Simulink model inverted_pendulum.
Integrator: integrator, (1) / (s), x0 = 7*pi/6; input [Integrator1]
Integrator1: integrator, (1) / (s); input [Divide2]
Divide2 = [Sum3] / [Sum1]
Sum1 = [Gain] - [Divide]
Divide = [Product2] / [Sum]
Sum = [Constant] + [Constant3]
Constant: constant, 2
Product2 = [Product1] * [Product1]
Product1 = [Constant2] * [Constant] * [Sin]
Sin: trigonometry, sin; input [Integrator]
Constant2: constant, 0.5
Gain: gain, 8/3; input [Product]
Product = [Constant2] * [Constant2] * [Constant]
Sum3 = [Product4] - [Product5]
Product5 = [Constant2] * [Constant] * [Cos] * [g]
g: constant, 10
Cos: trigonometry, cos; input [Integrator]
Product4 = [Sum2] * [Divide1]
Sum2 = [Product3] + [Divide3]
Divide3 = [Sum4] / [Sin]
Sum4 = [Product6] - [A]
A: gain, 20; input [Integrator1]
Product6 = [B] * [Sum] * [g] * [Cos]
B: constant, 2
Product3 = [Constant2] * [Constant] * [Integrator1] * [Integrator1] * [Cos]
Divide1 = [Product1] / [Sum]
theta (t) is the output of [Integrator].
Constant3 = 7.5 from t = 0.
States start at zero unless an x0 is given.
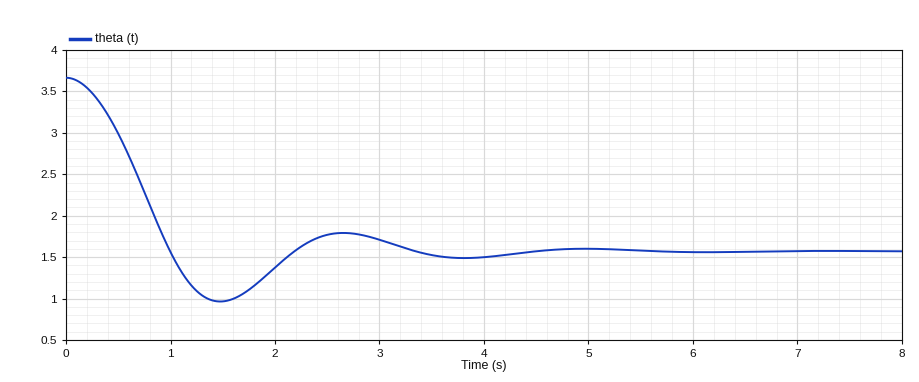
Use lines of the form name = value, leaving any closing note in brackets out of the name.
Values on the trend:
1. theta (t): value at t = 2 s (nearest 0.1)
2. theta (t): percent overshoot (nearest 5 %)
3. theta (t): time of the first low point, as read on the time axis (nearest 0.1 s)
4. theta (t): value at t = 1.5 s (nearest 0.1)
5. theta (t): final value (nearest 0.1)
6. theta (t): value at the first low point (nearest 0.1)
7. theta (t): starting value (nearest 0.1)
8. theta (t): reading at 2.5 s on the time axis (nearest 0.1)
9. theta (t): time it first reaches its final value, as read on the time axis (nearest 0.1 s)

theta (t): value at t = 2 s = 1.4
theta (t): percent overshoot = 30 %
theta (t): time of the first low point, as read on the time axis = 1.5 s
theta (t): value at t = 1.5 s = 1.0
theta (t): final value = 1.6
theta (t): value at the first low point = 1.0
theta (t): starting value = 3.7
theta (t): reading at 2.5 s on the time axis = 1.8
theta (t): time it first reaches its final value, as read on the time axis = 1.0 s
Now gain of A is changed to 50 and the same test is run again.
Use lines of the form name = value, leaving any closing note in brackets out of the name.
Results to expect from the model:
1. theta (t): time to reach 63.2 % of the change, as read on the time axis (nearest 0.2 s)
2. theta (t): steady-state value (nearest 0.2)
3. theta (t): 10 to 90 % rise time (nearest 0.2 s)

theta (t): time to reach 63.2 % of the change, as read on the time axis = 1.0 s
theta (t): steady-state value = 1.6
theta (t): 10 to 90 % rise time = 1.2 s
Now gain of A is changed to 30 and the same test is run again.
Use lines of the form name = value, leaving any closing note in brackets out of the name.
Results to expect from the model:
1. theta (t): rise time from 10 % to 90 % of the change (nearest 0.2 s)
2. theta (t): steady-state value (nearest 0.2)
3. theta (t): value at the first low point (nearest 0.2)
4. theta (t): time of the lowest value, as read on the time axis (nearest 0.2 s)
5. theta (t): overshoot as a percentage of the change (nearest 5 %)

theta (t): rise time from 10 % to 90 % of the change = 0.8 s
theta (t): steady-state value = 1.6
theta (t): value at the first low point = 1.2
theta (t): time of the lowest value, as read on the time axis = 1.6 s
theta (t): overshoot as a percentage of the change = 15 %
